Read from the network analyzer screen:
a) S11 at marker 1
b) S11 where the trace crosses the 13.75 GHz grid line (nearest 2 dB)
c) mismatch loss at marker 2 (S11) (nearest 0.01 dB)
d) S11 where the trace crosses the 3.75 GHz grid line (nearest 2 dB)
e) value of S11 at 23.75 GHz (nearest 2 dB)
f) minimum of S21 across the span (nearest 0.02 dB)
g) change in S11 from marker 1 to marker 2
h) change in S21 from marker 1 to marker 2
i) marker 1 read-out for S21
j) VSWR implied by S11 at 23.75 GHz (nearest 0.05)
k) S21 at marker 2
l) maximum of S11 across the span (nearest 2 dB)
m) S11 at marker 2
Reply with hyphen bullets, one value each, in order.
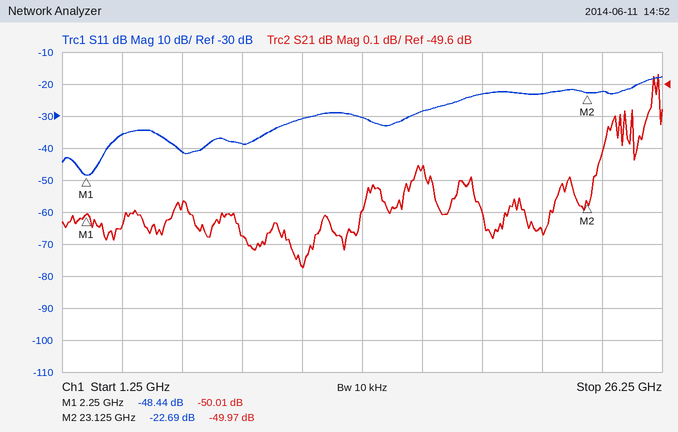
- -48.44 dB
- -30 dB
- 0.02 dB
- -36 dB
- -22 dB
- -50.18 dB
- 25.75 dB
- 0.04 dB
- -50.01 dB
- 1.15
- -49.97 dB
- -18 dB
- -22.69 dB
